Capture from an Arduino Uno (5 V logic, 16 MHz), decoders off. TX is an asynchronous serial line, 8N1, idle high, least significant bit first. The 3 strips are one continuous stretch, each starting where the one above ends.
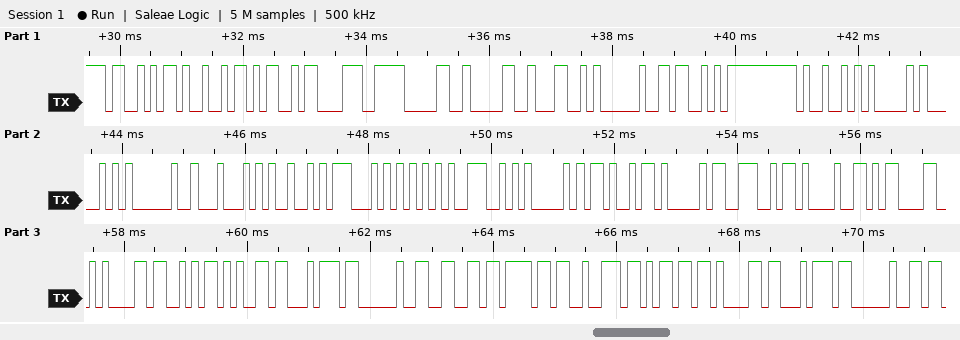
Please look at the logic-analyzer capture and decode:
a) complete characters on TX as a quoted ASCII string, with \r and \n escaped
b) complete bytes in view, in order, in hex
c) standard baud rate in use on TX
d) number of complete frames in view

"SIM800L SIAP DIGUNAKAN!\r\nSet format "
53 49 4D 38 30 30 4C 20 53 49 41 50 20 44 49 47 55 4E 41 4B 41 4E 21 0D 0A 53 65 74 20 66 6F 72 6D 61 74 20
9600 baud
36
